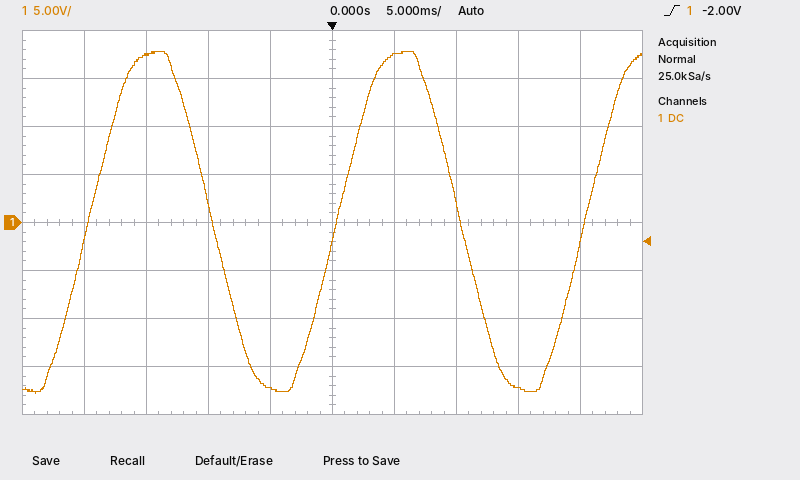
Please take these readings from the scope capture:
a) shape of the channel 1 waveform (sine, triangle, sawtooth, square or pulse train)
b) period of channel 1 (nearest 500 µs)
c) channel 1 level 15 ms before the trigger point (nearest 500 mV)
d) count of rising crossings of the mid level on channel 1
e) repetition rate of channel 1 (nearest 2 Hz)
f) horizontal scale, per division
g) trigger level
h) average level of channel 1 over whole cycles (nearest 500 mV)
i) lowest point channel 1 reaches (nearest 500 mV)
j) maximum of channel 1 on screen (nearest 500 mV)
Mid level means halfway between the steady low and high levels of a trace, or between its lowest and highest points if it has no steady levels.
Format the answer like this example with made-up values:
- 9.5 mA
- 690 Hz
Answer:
- sine
- 20.0 ms
- 17.5 V
- 3
- 50 Hz
- 5 ms
- -2.00 V
- 0.0 V
- -18.0 V
- 18.0 V
